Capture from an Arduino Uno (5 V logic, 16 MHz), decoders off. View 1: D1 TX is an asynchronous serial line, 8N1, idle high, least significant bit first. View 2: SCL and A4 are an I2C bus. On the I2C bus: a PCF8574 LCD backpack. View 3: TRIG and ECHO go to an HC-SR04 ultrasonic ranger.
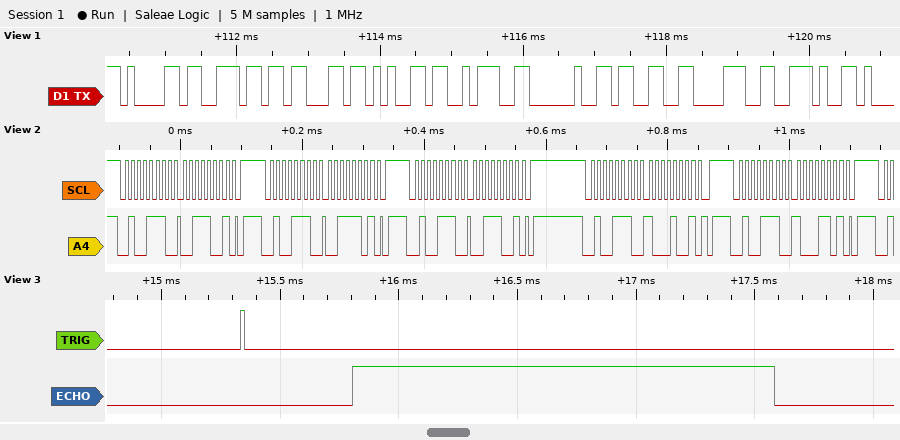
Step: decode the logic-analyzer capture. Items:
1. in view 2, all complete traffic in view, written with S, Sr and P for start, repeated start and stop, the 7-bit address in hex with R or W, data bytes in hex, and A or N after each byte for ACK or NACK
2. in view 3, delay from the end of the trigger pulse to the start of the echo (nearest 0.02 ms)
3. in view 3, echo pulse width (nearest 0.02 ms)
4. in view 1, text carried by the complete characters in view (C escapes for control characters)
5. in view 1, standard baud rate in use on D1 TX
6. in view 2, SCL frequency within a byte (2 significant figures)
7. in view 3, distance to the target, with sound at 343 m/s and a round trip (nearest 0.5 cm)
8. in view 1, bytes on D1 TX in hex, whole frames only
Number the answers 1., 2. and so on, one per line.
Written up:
1. S 27W A 39 A P S 27W A 3D A P S 27W A 39 A P S 27W A 89 A P S 27W A 8D A P
2. 0.46 ms
3. 1.78 ms
4. "ance: 38."
5. 9600 baud
6. 100 kHz
7. 30.5 cm
8. 0x61 0x6E 0x63 0x65 0x3A 0x20 0x33 0x38 0x2E
